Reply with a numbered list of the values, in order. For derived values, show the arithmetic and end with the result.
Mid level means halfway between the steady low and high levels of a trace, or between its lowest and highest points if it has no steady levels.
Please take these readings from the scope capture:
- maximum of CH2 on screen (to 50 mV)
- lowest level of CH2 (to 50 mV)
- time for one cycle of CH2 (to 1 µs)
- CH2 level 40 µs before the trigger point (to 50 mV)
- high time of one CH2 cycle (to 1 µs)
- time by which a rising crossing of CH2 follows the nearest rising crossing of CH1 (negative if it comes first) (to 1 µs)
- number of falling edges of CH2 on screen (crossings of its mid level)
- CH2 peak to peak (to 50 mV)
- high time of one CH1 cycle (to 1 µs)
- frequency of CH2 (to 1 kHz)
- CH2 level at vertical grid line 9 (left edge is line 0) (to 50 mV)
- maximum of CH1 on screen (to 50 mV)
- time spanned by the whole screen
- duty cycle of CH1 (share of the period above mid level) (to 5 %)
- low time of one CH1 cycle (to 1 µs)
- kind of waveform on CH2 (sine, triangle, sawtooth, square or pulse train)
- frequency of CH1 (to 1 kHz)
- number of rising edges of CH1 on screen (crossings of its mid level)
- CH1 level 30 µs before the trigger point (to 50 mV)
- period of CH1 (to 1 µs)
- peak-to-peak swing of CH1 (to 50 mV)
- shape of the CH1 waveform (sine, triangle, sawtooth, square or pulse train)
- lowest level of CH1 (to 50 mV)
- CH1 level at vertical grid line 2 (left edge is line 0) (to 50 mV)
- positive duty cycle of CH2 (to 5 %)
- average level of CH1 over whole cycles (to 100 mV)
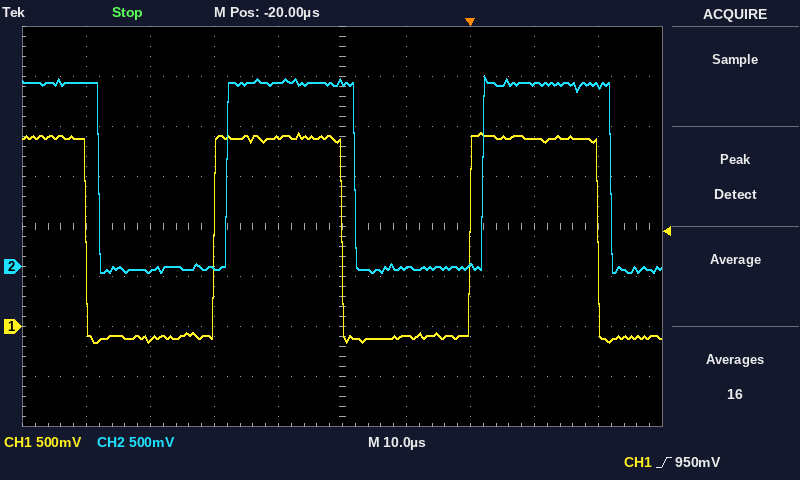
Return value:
1. 1.90 V
2. -50 mV
3. 40 µs
4. 0 mV
5. 20 µs
6. +2 µs
7. 3
8. 1.90 V − (-50 mV) = 1.95 V
9. 20 µs
10. 1 / 40 µs ≈ 25 kHz
11. 1.80 V
12. 1.95 V
13. 100 µs
14. 20 µs / 40 µs ≈ 50 %
15. 20 µs
16. square
17. 1 / 40 µs ≈ 25 kHz
18. 2
19. 1.90 V
20. 40 µs
21. 1.95 V − (-150 mV) = 2.10 V
22. square
23. -150 mV
24. -150 mV
25. 20 µs / 40 µs ≈ 50 %
26. -150 mV + 0.5 × (1.95 V − (-150 mV)) ≈ 900 mV
